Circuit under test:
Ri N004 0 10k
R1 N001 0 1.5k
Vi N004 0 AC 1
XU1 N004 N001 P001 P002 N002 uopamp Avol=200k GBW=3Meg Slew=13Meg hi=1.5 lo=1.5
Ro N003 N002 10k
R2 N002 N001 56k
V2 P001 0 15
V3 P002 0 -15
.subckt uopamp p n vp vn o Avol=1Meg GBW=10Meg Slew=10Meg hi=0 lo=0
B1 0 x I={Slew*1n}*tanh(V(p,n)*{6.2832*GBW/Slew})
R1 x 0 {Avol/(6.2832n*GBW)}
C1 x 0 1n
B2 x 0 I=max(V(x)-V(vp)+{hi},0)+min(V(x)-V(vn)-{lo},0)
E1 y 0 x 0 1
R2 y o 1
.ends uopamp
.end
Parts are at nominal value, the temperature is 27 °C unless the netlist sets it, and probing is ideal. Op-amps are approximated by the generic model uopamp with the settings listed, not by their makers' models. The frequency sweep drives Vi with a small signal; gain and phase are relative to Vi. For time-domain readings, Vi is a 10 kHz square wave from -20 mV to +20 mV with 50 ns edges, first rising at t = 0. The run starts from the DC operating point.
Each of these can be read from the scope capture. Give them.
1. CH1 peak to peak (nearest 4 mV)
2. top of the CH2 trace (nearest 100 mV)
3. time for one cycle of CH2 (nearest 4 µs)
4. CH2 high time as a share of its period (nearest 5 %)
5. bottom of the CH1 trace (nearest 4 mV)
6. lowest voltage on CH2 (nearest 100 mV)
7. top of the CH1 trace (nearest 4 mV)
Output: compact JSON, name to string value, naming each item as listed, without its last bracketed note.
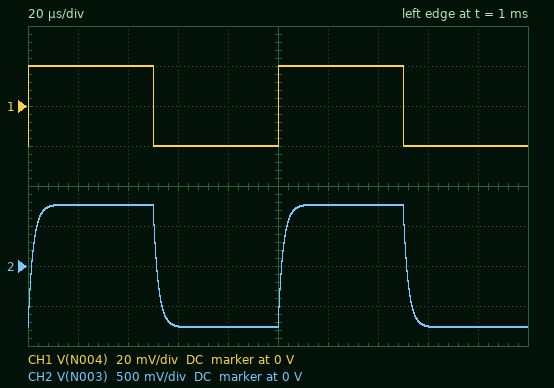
{"CH1 peak to peak": "40 mV", "top of the CH2 trace": "800 mV", "time for one cycle of CH2": "100 µs", "CH2 high time as a share of its period": "50 %", "bottom of the CH1 trace": "-20 mV", "lowest voltage on CH2": "-800 mV", "top of the CH1 trace": "20 mV"}
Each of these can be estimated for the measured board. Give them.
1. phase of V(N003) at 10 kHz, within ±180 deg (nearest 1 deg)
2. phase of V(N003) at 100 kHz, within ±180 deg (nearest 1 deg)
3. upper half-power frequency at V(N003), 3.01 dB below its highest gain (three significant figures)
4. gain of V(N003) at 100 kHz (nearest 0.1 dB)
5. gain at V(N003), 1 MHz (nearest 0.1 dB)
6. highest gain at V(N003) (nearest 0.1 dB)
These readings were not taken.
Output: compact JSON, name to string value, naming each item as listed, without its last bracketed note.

{"phase of V(N003) at 10 kHz, within ±180 deg": "-7 deg", "phase of V(N003) at 100 kHz, within ±180 deg": "-52 deg", "upper half-power frequency at V(N003), 3.01 dB below its highest gain": "78.3 kHz", "gain of V(N003) at 100 kHz": "27.5 dB", "gain at V(N003), 1 MHz": "9.5 dB", "highest gain at V(N003)": "31.7 dB"}
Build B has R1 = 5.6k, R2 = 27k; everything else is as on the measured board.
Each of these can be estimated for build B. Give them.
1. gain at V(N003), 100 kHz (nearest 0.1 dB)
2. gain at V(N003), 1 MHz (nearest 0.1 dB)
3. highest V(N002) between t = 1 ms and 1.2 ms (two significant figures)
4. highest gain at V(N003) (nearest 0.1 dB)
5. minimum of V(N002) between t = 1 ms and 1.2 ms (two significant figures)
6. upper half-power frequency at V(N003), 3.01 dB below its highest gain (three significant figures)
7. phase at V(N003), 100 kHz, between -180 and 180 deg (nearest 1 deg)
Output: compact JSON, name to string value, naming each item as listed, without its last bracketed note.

{"gain at V(N003), 100 kHz": "15.1 dB", "gain at V(N003), 1 MHz": "8.5 dB", "highest V(N002) between t = 1 ms and 1.2 ms": "120 mV", "highest gain at V(N003)": "15.3 dB", "minimum of V(N002) between t = 1 ms and 1.2 ms": "-120 mV", "upper half-power frequency at V(N003), 3.01 dB below its highest gain": "515 kHz", "phase at V(N003), 100 kHz, between -180 and 180 deg": "-11 deg"}
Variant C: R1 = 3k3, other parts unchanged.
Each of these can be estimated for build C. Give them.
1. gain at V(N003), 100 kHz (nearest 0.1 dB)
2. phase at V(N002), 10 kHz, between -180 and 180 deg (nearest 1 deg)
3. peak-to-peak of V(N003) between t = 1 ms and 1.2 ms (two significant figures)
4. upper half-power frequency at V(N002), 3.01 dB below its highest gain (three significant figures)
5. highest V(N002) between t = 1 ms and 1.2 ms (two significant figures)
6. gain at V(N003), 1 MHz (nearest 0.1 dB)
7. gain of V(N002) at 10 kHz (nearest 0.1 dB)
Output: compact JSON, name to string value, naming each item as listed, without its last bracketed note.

{"gain at V(N003), 100 kHz": "23.8 dB", "phase at V(N002), 10 kHz, between -180 and 180 deg": "-3 deg", "peak-to-peak of V(N003) between t = 1 ms and 1.2 ms": "720 mV", "upper half-power frequency at V(N002), 3.01 dB below its highest gain": "167 kHz", "highest V(N002) between t = 1 ms and 1.2 ms": "360 mV", "gain at V(N003), 1 MHz": "9.4 dB", "gain of V(N002) at 10 kHz": "25.1 dB"}
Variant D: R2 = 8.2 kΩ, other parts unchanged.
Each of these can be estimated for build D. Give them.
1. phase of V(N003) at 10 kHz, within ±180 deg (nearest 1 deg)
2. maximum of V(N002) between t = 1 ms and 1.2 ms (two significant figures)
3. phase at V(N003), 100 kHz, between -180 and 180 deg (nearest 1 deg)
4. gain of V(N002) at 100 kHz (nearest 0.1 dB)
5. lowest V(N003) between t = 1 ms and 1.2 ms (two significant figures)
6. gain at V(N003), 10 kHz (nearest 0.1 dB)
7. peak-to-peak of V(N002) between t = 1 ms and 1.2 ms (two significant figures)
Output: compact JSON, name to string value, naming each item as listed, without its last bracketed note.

{"phase of V(N003) at 10 kHz, within ±180 deg": "-1 deg", "maximum of V(N002) between t = 1 ms and 1.2 ms": "130 mV", "phase at V(N003), 100 kHz, between -180 and 180 deg": "-12 deg", "gain of V(N002) at 100 kHz": "16.0 dB", "lowest V(N003) between t = 1 ms and 1.2 ms": "-130 mV", "gain at V(N003), 10 kHz": "16.2 dB", "peak-to-peak of V(N002) between t = 1 ms and 1.2 ms": "260 mV"}
